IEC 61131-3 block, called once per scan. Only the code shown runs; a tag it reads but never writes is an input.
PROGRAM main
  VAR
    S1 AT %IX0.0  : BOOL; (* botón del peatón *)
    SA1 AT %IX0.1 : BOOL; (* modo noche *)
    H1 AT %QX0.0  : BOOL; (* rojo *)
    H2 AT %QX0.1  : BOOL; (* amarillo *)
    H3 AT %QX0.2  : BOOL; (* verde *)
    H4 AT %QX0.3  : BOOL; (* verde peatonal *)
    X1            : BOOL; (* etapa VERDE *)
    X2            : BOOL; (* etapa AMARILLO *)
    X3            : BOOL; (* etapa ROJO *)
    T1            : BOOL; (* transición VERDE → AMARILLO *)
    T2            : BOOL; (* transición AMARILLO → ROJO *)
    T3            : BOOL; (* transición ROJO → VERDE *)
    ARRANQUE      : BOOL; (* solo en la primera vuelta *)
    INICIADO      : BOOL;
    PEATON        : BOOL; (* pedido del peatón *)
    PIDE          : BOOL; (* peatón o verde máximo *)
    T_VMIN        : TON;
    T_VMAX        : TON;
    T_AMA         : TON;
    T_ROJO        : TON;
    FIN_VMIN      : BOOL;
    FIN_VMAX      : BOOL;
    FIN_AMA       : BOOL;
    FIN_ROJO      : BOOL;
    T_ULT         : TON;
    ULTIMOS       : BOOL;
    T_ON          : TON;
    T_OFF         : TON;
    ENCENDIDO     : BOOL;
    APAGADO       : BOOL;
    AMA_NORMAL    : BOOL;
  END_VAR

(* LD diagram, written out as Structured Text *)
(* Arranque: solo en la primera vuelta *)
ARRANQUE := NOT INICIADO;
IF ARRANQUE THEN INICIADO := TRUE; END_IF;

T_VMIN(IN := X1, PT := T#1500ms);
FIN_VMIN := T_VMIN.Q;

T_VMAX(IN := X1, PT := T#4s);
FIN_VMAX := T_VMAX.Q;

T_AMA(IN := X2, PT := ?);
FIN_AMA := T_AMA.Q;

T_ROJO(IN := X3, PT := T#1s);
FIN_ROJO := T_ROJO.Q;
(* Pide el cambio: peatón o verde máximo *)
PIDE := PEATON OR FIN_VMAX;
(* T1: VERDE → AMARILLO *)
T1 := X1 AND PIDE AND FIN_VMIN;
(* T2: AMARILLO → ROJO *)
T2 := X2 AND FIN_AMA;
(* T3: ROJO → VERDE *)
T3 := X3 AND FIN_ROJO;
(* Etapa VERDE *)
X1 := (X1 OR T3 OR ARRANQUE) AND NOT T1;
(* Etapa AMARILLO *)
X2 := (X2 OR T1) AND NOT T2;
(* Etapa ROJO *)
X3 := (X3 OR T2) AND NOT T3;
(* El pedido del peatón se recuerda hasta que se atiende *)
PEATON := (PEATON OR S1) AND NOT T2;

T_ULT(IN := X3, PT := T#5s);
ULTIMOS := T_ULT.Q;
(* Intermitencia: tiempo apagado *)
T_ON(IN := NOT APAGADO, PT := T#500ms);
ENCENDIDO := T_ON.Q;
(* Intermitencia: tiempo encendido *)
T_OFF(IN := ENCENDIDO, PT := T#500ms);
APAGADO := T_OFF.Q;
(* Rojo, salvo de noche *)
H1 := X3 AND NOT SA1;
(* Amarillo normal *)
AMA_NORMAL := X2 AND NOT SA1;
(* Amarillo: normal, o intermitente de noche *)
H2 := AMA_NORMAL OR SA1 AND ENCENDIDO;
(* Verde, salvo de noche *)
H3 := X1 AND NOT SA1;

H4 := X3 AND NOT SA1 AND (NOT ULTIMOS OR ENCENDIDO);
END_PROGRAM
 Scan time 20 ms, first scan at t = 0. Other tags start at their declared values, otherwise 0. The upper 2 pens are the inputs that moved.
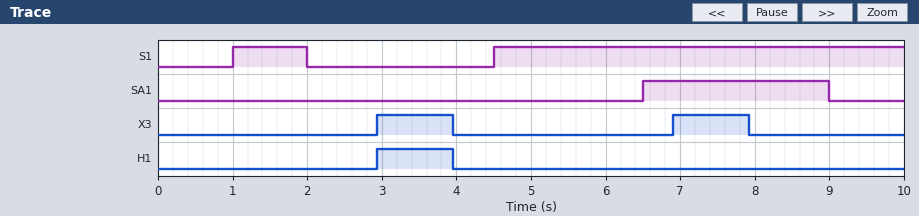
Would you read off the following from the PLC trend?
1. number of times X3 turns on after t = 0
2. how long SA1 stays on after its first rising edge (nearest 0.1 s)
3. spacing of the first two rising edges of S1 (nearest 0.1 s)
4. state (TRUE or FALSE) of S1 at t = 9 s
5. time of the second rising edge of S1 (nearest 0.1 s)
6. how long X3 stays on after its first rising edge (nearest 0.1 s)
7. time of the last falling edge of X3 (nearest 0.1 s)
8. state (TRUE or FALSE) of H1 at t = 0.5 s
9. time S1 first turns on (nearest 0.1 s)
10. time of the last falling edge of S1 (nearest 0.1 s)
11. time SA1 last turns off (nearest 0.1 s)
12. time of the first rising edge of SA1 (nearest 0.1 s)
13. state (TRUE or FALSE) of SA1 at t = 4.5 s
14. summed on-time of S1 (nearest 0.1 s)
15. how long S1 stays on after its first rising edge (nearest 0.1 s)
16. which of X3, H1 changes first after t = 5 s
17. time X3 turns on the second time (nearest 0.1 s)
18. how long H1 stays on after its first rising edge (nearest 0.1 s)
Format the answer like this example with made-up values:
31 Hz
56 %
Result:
2
2.5 s
3.5 s
TRUE
4.5 s
1.0 s
7.9 s
FALSE
1.0 s
2.0 s
9.0 s
6.5 s
FALSE
6.5 s
1.0 s
X3
6.9 s
1.0 s
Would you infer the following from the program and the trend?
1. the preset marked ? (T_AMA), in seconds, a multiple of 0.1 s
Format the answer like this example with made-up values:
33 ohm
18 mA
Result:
1.4 s
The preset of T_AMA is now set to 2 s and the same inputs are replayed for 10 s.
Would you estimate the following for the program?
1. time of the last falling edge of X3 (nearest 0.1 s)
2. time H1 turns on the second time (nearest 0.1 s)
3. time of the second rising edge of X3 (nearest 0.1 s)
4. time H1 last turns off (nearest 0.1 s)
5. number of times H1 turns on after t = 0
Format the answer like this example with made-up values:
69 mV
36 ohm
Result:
9.1 s
9.0 s
8.1 s
9.1 s
2
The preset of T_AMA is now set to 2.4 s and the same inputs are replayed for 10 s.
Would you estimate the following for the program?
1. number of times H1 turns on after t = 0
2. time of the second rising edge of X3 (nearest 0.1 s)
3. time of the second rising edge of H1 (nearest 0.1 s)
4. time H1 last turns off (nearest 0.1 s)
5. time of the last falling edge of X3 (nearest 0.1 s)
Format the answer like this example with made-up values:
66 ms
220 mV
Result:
2
8.9 s
9.0 s
9.9 s
9.9 s
